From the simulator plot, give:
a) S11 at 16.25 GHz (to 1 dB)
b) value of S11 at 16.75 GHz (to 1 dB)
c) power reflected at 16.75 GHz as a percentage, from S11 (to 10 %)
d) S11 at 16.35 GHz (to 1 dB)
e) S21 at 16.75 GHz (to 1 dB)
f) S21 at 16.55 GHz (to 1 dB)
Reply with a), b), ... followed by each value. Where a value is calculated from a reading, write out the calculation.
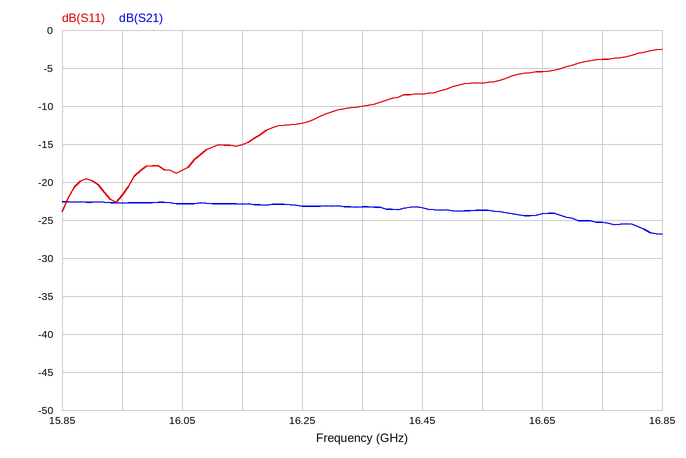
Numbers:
a) -12 dB
b) -4 dB
c) 10^(-4/10) ≈ 40 %
d) -10 dB
e) -25 dB
f) -24 dB
